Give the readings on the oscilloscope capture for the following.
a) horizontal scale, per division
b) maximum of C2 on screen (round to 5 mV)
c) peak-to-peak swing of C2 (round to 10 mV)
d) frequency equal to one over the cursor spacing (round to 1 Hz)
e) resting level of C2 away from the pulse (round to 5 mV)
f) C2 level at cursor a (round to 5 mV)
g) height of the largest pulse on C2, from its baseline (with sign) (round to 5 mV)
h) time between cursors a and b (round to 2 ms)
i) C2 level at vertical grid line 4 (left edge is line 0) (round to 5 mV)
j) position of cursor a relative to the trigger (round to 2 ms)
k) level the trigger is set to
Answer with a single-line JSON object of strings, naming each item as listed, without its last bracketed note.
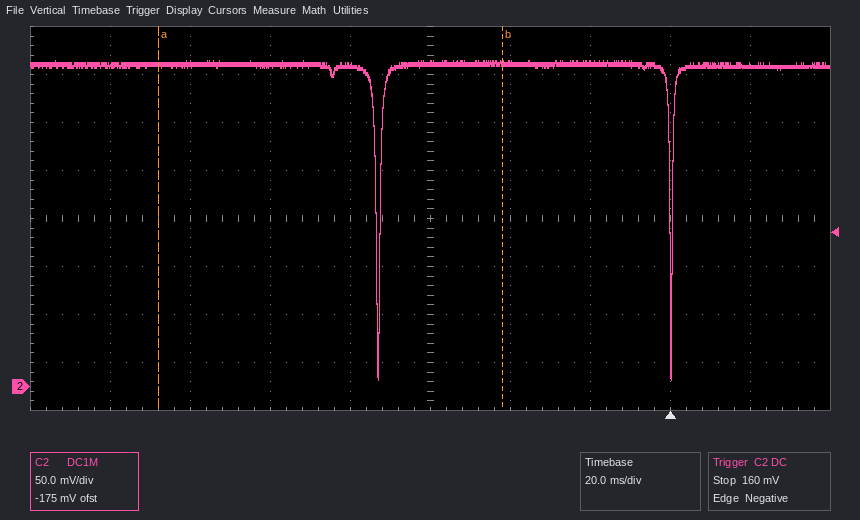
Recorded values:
{"horizontal scale, per division": "20 ms", "maximum of C2 on screen": "340 mV", "peak-to-peak swing of C2": "330 mV", "frequency equal to one over the cursor spacing": "12 Hz", "resting level of C2 away from the pulse": "335 mV", "C2 level at cursor a": "335 mV", "height of the largest pulse on C2, from its baseline (with sign)": "-330 mV", "time between cursors a and b": "86 ms", "C2 level at vertical grid line 4 (left edge is line 0)": "335 mV", "position of cursor a relative to the trigger": "-128 ms", "level the trigger is set to": "160 mV"}
